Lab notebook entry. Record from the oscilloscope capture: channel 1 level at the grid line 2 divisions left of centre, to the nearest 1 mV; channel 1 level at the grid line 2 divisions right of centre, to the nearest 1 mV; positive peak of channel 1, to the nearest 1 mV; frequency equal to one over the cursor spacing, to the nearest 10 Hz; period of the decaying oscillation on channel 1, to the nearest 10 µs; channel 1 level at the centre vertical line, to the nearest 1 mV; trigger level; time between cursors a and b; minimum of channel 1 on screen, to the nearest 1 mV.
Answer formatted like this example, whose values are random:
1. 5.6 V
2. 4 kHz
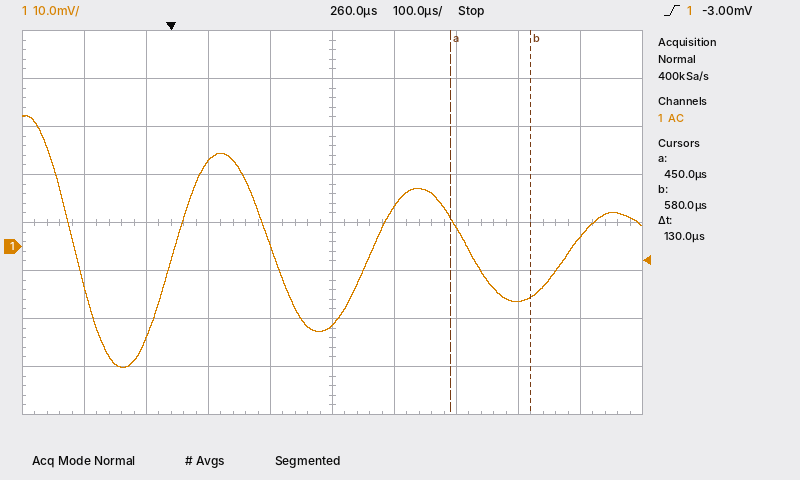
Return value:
1. 18 mV
2. 4 mV
3. 27 mV
4. 7.69 kHz
5. 320 µs
6. -16 mV
7. -3.00 mV
8. 130 µs
9. -25 mV
